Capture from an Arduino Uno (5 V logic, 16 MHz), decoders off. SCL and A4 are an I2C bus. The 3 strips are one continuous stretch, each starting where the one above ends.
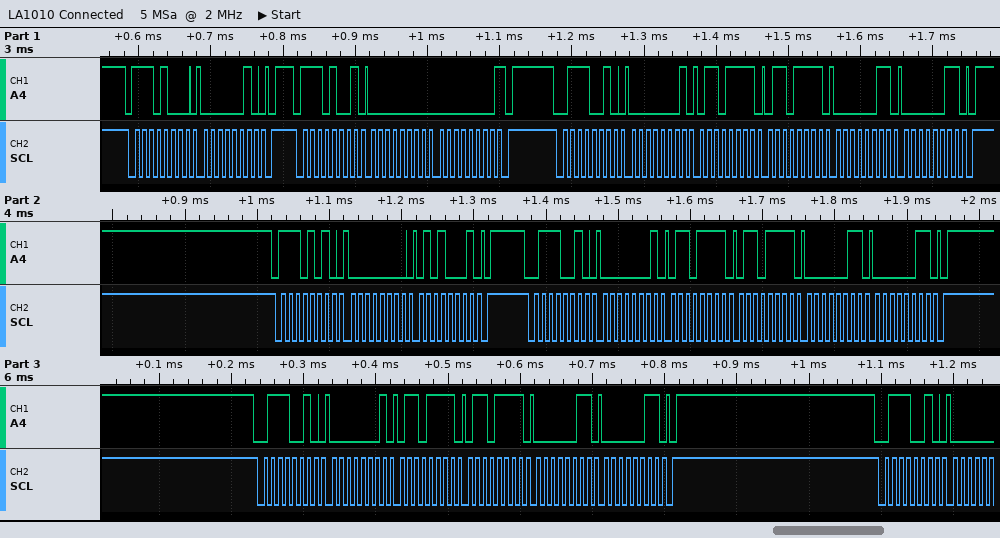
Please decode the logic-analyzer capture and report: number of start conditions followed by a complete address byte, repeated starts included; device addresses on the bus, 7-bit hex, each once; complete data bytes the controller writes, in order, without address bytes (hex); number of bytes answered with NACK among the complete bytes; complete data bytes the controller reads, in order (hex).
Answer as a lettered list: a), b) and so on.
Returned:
a) 7
b) 0x74 0x39 0x75
c) 02 01 6F 6F 03 03 00 51 01 6F 6F 03 03 01 6F 6F 03 03
d) 1
e) 00 00
